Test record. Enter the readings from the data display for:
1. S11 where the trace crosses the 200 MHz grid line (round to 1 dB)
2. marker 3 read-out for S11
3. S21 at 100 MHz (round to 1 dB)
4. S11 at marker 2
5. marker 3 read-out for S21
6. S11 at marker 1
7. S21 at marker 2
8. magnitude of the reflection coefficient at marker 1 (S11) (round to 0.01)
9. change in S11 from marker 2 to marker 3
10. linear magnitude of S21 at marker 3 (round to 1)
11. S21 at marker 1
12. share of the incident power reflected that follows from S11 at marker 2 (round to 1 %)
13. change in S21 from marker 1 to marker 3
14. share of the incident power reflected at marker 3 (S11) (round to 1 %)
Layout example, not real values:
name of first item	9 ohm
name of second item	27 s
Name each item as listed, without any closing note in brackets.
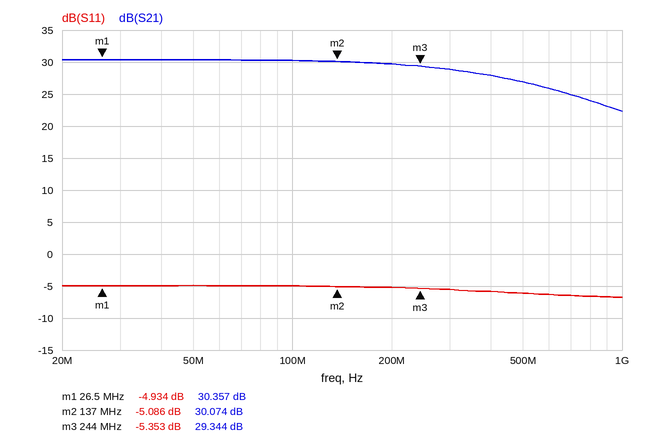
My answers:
S11 where the trace crosses the 200 MHz grid line	-5 dB
marker 3 read-out for S11	-5.353 dB
S21 at 100 MHz	30 dB
S11 at marker 2	-5.086 dB
marker 3 read-out for S21	29.344 dB
S11 at marker 1	-4.934 dB
S21 at marker 2	30.074 dB
magnitude of the reflection coefficient at marker 1 (S11)	0.57
change in S11 from marker 2 to marker 3	-0.267 dB
linear magnitude of S21 at marker 3	29
S21 at marker 1	30.357 dB
share of the incident power reflected that follows from S11 at marker 2	31 %
change in S21 from marker 1 to marker 3	-1.013 dB
share of the incident power reflected at marker 3 (S11)	29 %
